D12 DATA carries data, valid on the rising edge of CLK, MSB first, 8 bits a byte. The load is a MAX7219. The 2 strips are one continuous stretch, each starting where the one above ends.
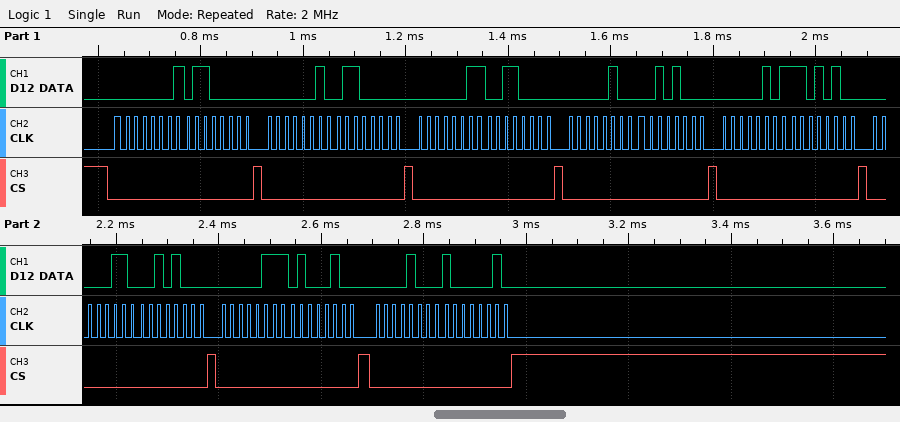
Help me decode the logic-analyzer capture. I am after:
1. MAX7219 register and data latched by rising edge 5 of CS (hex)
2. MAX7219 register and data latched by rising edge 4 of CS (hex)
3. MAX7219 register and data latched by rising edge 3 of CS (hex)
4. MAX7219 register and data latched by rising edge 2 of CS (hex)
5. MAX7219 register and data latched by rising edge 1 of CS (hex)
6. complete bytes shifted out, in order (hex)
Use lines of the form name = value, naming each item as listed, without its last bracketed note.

MAX7219 register and data latched by rising edge 5 of CS = register 0x5, data 0xD4
MAX7219 register and data latched by rising edge 4 of CS = register 0x4, data 0x28
MAX7219 register and data latched by rising edge 3 of CS = register 0x3, data 0x30
MAX7219 register and data latched by rising edge 2 of CS = register 0x2, data 0x60
MAX7219 register and data latched by rising edge 1 of CS = register 0x1, data 0x60
complete bytes shifted out, in order = 01 60 02 60 03 30 04 28 05 D4 06 28 07 44 08 82
